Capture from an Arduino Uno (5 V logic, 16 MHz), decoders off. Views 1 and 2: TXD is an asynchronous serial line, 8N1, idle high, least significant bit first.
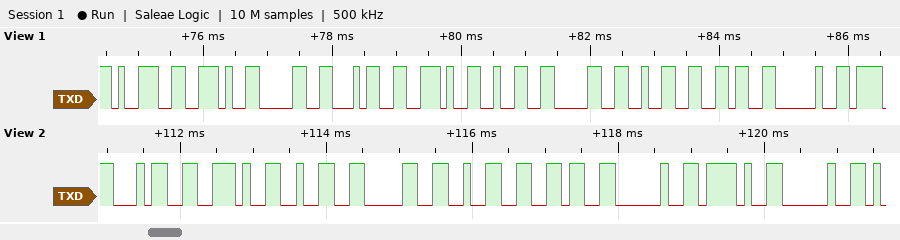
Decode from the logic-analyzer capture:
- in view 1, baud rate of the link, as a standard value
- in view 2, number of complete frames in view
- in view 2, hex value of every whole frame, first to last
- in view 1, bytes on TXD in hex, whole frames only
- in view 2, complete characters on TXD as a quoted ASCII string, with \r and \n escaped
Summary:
9600 baud
9
34 2E 32 30 32 36 20 2F 20
39 2E 30 34 2E 32 30 32 36 20
"4.2026 / "
